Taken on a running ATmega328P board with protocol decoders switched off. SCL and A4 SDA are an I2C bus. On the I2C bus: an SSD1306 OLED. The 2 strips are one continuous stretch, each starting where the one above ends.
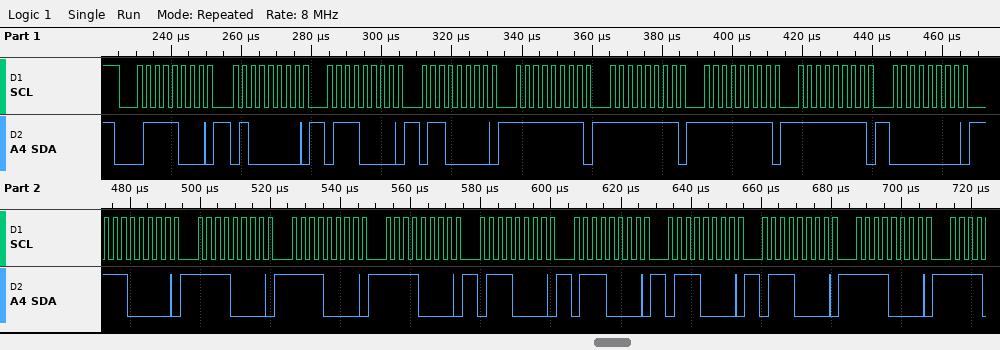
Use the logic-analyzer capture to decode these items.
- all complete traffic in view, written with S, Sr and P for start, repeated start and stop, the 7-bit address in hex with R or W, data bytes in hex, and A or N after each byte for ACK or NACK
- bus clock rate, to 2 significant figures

S 3CW A 40 A 70 A 60 A FF A FF A FF A FF A 00 A E0 A F0 A F0 A F0 A 70 A 70 A 70 A 70 A F0 A
400 kHz
